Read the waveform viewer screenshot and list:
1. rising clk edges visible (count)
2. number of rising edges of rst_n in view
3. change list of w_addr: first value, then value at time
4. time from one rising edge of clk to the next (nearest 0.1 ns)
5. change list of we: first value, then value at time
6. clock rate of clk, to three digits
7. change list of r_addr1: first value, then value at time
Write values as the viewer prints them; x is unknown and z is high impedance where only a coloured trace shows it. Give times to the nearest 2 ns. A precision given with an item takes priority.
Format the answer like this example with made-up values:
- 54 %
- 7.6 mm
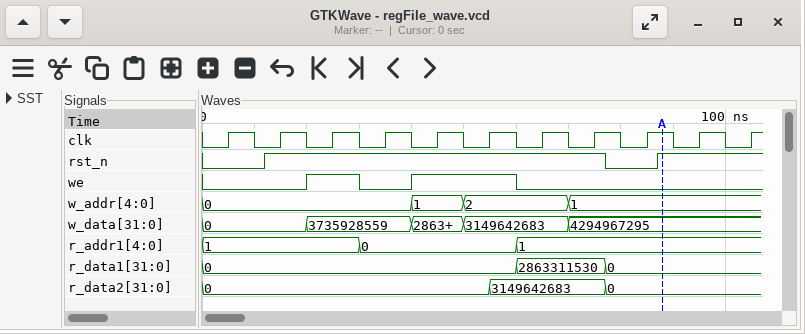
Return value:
- 11
- 2
- 0, 1 at 40 ns, 2 at 50 ns, 1 at 70 ns
- 10 ns
- 0, 1 at 20 ns, 0 at 30 ns, 1 at 40 ns, 0 at 60 ns
- 100 MHz
- 1, 0 at 30 ns, 1 at 60 ns
